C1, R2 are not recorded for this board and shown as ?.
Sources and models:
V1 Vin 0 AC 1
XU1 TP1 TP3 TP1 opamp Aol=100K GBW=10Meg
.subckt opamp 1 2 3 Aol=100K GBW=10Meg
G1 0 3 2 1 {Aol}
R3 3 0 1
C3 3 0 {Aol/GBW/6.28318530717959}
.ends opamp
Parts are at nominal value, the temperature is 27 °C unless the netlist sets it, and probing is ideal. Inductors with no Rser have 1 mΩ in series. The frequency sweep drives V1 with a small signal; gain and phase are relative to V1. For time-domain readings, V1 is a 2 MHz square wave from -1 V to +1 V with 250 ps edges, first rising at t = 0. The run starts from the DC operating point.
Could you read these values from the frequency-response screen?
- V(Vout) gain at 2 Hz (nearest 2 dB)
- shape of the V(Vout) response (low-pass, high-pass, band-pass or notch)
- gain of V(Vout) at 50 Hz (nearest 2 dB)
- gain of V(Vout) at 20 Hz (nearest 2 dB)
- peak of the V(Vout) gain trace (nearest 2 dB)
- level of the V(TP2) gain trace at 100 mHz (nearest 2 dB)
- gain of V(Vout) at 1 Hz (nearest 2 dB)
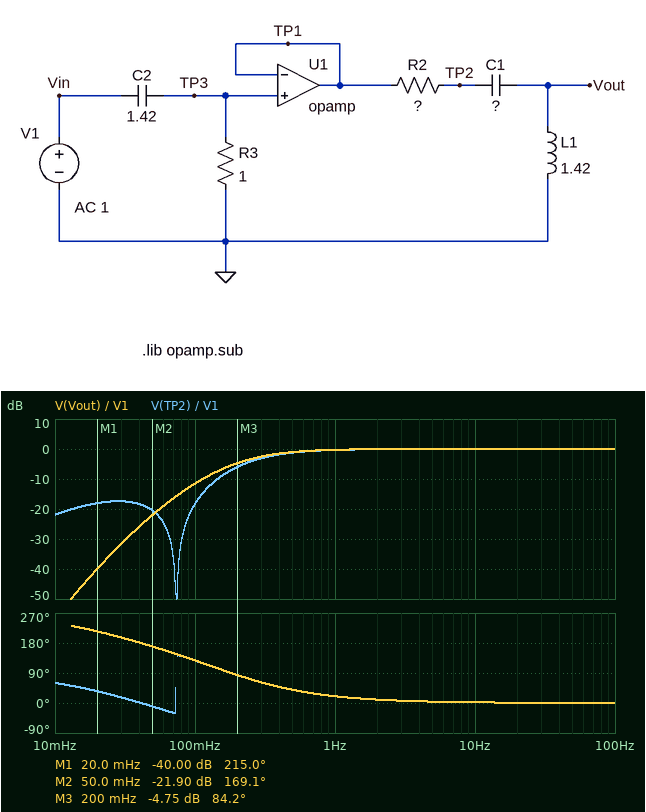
0 dB
high-pass
0 dB
0 dB
0 dB
-18 dB
0 dB
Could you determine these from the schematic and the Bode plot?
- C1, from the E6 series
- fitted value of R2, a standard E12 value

3.3 F
2.2 Ω
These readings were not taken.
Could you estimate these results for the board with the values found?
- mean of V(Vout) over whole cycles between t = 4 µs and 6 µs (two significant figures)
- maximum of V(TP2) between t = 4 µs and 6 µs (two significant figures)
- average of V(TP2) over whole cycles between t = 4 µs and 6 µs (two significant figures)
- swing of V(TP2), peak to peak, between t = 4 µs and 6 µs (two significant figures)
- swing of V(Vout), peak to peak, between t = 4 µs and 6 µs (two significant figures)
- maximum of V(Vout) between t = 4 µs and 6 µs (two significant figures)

1.0 V
2.0 V
1.0 V
2.0 V
2.0 V
2.0 V
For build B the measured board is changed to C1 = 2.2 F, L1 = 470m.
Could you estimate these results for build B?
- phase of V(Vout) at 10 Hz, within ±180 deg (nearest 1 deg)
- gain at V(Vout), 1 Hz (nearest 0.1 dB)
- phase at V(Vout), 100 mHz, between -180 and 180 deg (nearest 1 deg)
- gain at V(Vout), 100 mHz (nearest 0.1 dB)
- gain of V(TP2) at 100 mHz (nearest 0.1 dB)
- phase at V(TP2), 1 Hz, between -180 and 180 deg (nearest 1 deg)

5 deg
-1.8 dB
149 deg
-21.1 dB
-17.9 dB
44 deg
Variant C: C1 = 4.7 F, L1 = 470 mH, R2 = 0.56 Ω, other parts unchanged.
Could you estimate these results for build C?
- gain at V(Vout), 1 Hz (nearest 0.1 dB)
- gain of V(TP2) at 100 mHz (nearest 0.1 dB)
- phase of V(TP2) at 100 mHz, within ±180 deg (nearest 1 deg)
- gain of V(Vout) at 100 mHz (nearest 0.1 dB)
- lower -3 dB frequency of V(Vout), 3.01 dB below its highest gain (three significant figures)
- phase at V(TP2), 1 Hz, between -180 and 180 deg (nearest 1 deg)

-0.1 dB
-25.8 dB
-36 deg
-9.1 dB
188 mHz
17 deg
